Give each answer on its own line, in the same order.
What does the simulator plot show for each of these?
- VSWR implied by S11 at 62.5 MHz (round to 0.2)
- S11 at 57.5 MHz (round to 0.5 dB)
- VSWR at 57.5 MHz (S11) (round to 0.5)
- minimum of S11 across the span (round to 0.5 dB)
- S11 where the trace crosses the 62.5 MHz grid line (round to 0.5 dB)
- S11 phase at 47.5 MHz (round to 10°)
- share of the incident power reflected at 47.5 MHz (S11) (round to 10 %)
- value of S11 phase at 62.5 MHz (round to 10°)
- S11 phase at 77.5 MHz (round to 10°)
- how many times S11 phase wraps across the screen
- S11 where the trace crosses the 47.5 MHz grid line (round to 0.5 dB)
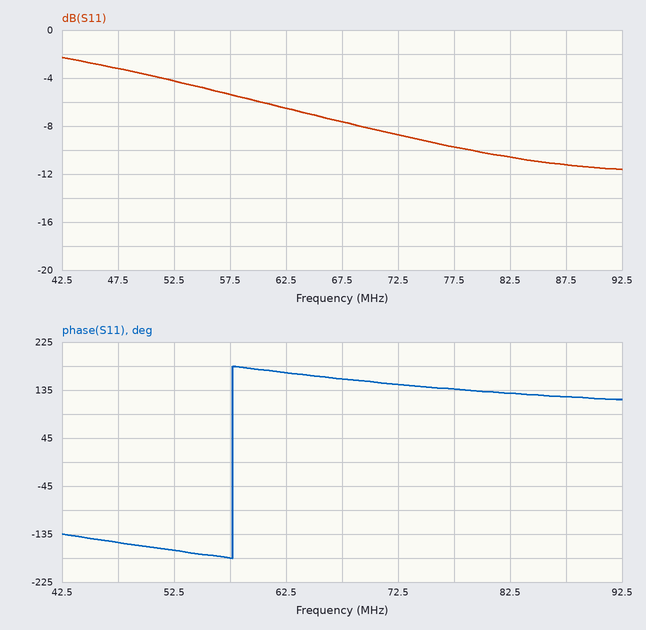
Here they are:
2.8
-5.5 dB
3.5
-11.5 dB
-6.5 dB
-150°
50 %
170°
140°
1
-3.0 dB
